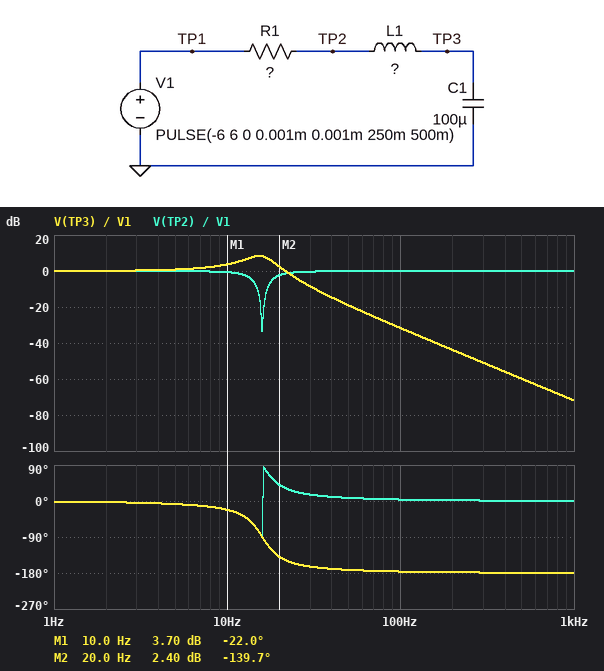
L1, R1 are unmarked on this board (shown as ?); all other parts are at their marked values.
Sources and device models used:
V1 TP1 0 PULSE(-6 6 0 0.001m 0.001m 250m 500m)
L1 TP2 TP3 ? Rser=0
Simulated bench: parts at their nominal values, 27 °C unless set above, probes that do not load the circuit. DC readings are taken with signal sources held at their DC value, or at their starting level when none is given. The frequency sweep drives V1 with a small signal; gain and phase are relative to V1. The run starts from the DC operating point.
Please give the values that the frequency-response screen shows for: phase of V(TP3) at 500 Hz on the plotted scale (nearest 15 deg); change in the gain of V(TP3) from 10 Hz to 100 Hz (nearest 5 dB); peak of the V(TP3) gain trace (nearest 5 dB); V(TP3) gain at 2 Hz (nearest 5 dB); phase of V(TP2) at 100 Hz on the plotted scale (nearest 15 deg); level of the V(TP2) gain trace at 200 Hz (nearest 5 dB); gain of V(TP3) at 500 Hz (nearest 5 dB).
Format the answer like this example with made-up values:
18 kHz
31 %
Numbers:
-180 deg
-35 dB
10 dB
0 dB
0 deg
0 dB
-60 dB
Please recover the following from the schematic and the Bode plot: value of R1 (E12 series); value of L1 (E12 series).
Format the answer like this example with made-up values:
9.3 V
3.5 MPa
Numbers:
39 Ω
1 H
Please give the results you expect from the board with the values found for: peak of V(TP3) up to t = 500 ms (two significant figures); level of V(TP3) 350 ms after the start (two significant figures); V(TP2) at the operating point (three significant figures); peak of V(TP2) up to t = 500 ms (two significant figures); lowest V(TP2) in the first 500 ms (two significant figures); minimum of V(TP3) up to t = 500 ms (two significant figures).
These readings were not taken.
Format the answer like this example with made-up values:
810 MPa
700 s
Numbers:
12 V
-7.7 V
-6.00 V
7.9 V
-7.9 V
-12 V
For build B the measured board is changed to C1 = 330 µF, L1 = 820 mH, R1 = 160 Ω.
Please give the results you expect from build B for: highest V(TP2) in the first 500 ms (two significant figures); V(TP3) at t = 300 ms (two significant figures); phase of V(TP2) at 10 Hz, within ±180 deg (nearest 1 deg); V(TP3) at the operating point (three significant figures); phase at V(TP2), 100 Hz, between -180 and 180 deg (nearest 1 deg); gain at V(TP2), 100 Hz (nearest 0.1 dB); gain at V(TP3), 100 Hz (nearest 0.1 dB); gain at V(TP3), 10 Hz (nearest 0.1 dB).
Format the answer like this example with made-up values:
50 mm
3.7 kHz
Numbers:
6.1 V
-1.3 V
89 deg
-6.00 V
17 deg
-0.4 dB
-40.9 dB
-10.4 dB
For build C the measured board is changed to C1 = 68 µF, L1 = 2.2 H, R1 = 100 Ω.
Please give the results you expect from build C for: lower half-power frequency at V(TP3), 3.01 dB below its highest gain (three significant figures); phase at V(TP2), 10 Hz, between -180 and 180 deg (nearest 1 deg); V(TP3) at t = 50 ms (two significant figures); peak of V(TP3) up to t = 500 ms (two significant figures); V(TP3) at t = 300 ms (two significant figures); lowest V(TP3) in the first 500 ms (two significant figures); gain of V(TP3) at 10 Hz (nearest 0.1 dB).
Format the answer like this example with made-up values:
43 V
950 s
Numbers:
7.26 Hz
-46 deg
9.5 V
11 V
-9.5 V
-11 V
4.6 dB
